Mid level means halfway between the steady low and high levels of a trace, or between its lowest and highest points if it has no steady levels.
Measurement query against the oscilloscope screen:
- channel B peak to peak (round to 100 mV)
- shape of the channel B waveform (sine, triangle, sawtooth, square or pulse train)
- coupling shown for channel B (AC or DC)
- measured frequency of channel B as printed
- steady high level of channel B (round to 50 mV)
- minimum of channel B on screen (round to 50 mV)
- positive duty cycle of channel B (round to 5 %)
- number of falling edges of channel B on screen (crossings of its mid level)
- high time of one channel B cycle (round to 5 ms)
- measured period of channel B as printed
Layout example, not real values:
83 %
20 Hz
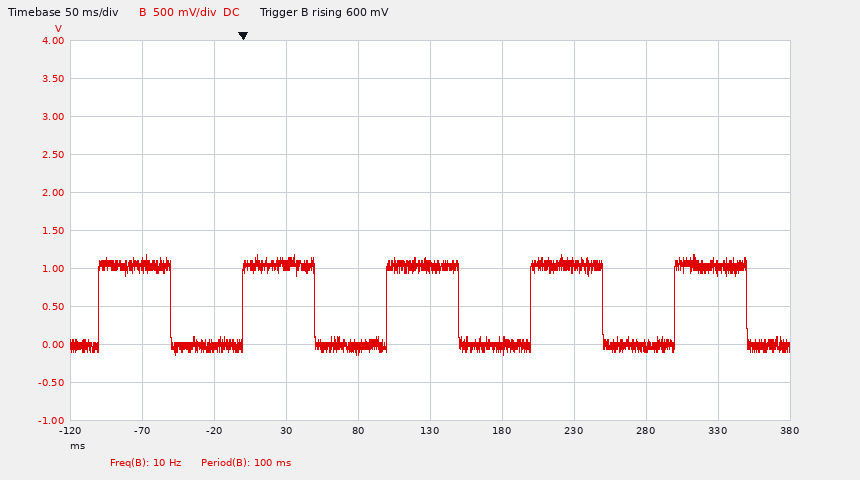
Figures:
1.30 V
square
DC
10 Hz
1.05 V
-150 mV
50 %
5
50 ms
100 ms
